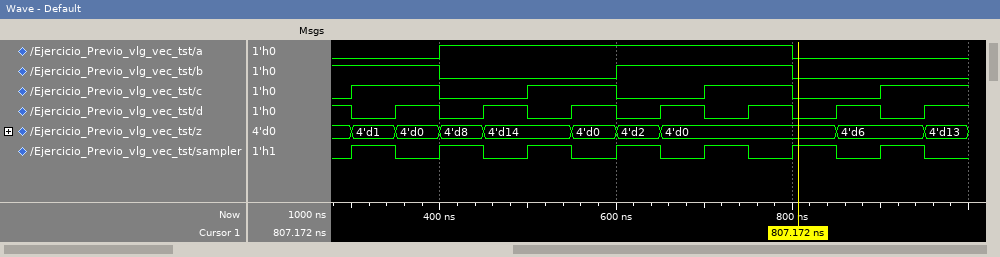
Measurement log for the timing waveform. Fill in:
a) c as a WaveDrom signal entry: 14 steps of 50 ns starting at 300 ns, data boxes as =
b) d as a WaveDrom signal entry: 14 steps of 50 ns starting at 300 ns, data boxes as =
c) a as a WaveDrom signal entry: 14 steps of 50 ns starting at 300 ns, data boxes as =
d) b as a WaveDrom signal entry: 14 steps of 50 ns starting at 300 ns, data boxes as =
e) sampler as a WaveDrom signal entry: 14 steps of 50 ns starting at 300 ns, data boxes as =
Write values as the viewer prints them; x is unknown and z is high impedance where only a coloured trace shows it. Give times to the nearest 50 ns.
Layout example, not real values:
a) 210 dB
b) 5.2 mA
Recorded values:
a) {name: 'c', wave: '1.0.1.0.1.0.1.'}
b) {name: 'd', wave: '01010101010101'}
c) {name: 'a', wave: '0.1.......0...'}
d) {name: 'b', wave: '1.0...1...0...'}
e) {name: 'sampler', wave: '10101010101010'}
